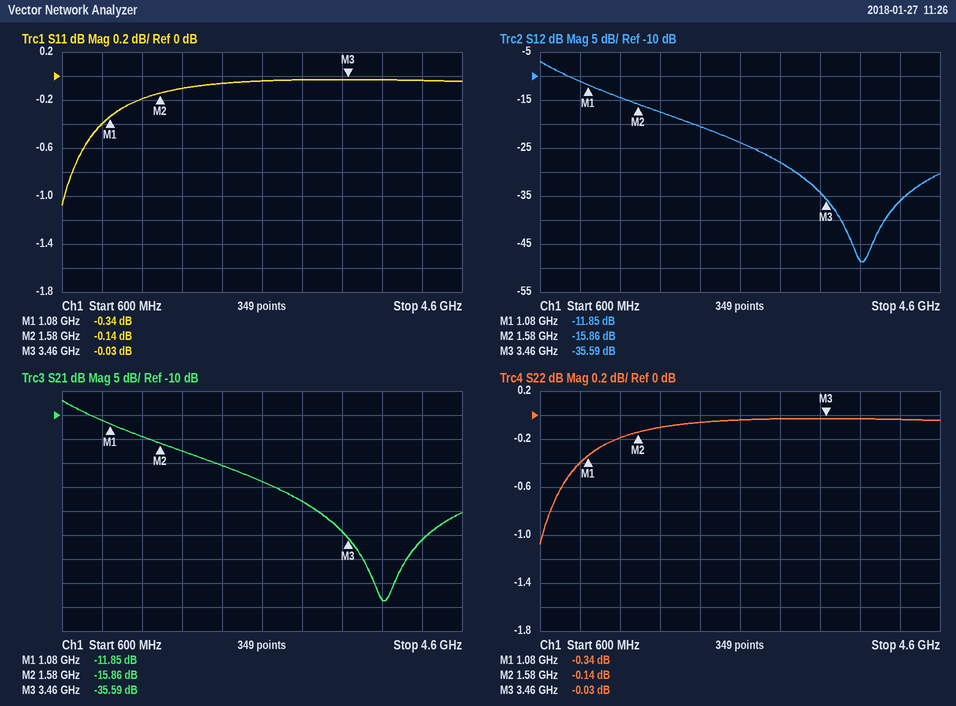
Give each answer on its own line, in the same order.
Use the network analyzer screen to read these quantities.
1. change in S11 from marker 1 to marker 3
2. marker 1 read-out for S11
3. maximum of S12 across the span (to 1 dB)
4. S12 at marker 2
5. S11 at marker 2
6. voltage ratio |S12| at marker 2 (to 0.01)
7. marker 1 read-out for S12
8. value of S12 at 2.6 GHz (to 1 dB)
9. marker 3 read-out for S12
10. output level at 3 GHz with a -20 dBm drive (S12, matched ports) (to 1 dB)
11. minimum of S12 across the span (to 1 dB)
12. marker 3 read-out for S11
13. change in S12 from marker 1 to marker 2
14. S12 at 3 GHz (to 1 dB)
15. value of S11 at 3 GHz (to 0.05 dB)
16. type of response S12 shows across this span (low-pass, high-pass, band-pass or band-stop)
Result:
0.31 dB
-0.34 dB
-7 dB
-15.86 dB
-0.14 dB
0.16
-11.85 dB
-24 dB
-35.59 dB
-48 dBm
-49 dB
-0.03 dB
-4.01 dB
-28 dB
-0.05 dB
low-pass
